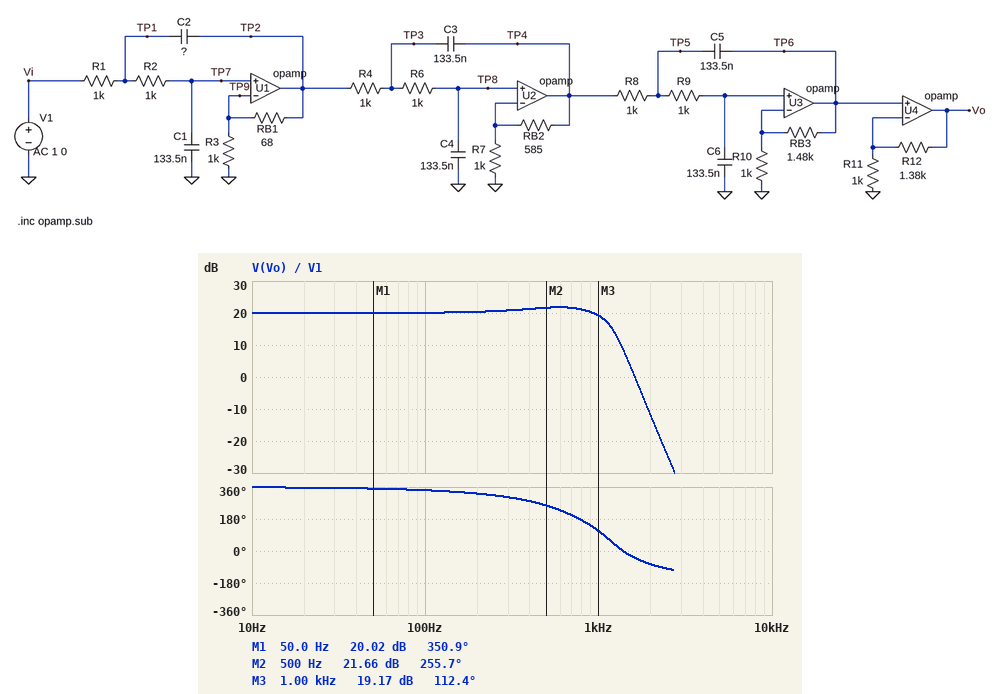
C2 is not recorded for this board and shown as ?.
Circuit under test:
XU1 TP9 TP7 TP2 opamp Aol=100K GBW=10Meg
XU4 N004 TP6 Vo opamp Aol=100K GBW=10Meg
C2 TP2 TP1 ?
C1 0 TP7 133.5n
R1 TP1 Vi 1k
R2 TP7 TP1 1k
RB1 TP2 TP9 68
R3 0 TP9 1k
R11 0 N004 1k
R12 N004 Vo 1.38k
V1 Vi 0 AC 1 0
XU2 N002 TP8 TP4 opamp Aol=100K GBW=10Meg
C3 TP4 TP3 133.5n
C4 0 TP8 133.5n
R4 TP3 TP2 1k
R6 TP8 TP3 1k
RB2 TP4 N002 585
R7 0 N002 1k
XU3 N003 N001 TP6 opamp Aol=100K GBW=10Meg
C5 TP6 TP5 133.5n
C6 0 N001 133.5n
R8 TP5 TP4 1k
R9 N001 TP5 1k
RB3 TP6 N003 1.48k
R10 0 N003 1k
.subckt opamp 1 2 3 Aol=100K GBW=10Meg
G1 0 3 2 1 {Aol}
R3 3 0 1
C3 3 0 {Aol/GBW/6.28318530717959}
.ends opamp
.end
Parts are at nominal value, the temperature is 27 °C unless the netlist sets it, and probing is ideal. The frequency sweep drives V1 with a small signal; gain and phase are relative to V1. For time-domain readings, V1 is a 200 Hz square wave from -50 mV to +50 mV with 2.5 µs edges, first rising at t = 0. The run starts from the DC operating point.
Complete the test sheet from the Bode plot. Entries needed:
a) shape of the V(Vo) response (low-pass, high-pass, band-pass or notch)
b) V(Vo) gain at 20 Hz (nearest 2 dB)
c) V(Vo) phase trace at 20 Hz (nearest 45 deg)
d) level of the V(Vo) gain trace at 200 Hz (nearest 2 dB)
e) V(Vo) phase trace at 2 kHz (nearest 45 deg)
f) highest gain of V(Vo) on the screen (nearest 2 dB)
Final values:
low-pass
20 dB
360 deg
20 dB
-90 deg
22 dB
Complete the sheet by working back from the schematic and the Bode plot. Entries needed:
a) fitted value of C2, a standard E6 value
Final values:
330 nF
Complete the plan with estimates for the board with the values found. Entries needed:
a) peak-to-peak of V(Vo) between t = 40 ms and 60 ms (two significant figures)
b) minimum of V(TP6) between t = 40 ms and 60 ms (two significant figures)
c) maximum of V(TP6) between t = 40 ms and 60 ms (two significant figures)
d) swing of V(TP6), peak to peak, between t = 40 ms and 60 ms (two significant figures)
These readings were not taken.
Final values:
1.5 V
-320 mV
320 mV
640 mV
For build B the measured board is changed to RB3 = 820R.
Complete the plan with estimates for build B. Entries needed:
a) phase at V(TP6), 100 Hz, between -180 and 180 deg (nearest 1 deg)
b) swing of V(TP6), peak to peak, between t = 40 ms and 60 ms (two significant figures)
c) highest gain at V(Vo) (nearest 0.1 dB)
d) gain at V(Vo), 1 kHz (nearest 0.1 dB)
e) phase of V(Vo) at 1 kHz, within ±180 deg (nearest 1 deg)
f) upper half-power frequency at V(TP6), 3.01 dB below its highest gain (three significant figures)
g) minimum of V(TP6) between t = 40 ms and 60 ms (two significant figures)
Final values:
-21 deg
400 mV
18.0 dB
10.6 dB
95 deg
801 Hz
-200 mV
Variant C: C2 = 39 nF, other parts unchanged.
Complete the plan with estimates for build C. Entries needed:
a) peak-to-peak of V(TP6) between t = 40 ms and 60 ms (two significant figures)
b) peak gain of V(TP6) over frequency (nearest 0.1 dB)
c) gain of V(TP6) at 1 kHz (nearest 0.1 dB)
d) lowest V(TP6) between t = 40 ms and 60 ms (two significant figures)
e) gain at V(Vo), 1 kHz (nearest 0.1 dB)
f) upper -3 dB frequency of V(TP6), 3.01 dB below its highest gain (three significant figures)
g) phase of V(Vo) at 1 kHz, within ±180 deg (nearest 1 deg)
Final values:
480 mV
12.5 dB
11.0 dB
-240 mV
18.5 dB
1.15 kHz
164 deg
